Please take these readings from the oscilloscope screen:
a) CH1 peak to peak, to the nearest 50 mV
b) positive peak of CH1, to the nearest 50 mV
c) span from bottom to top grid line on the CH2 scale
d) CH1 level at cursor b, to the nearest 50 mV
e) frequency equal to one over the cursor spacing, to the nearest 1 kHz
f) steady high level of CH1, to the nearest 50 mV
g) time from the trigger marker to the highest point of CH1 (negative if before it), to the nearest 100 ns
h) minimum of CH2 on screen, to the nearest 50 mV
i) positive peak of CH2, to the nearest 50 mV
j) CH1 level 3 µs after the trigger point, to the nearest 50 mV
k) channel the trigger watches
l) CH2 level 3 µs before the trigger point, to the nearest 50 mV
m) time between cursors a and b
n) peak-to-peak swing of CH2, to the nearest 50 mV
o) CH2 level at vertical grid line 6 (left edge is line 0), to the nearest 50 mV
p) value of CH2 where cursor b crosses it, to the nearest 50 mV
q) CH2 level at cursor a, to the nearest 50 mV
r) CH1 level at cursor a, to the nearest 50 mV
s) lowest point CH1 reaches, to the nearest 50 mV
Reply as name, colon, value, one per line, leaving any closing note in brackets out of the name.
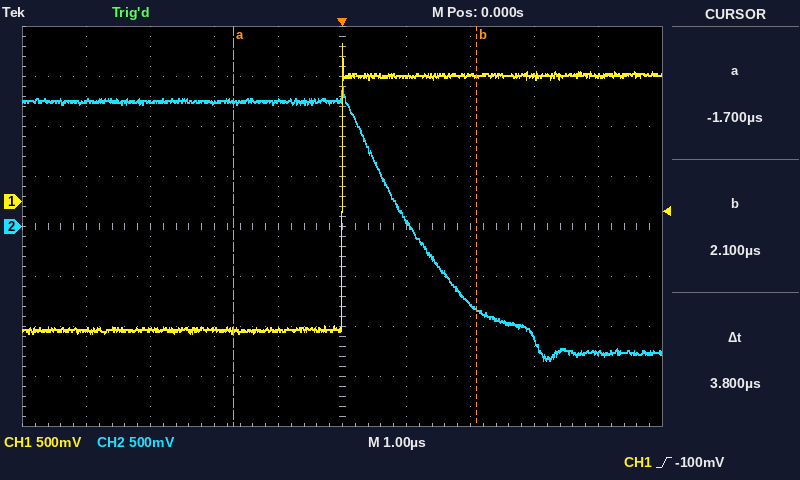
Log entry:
CH1 peak to peak, to the nearest 50 mV: 2.90 V
positive peak of CH1, to the nearest 50 mV: 1.60 V
span from bottom to top grid line on the CH2 scale: 4 V
CH1 level at cursor b, to the nearest 50 mV: 1.25 V
frequency equal to one over the cursor spacing, to the nearest 1 kHz: 263 kHz
steady high level of CH1, to the nearest 50 mV: 1.25 V
time from the trigger marker to the highest point of CH1 (negative if before it), to the nearest 100 ns: 0.0 µs
minimum of CH2 on screen, to the nearest 50 mV: -1.35 V
positive peak of CH2, to the nearest 50 mV: 1.40 V
CH1 level 3 µs after the trigger point, to the nearest 50 mV: 1.25 V
channel the trigger watches: CH1
CH2 level 3 µs before the trigger point, to the nearest 50 mV: 1.25 V
time between cursors a and b: 3.8 µs
peak-to-peak swing of CH2, to the nearest 50 mV: 2.75 V
CH2 level at vertical grid line 6 (left edge is line 0), to the nearest 50 mV: 50 mV
value of CH2 where cursor b crosses it, to the nearest 50 mV: -850 mV
CH2 level at cursor a, to the nearest 50 mV: 1.25 V
CH1 level at cursor a, to the nearest 50 mV: -1.30 V
lowest point CH1 reaches, to the nearest 50 mV: -1.30 V
